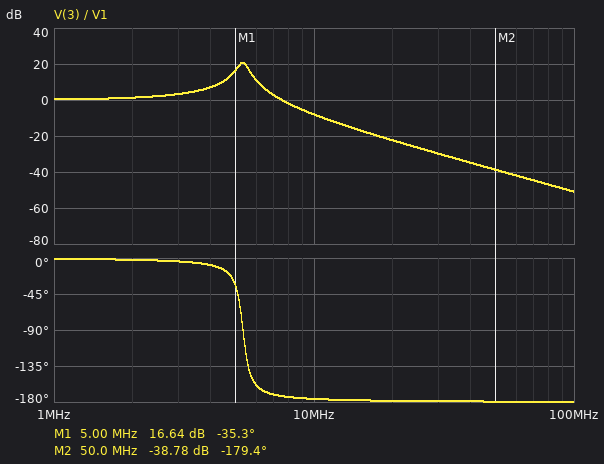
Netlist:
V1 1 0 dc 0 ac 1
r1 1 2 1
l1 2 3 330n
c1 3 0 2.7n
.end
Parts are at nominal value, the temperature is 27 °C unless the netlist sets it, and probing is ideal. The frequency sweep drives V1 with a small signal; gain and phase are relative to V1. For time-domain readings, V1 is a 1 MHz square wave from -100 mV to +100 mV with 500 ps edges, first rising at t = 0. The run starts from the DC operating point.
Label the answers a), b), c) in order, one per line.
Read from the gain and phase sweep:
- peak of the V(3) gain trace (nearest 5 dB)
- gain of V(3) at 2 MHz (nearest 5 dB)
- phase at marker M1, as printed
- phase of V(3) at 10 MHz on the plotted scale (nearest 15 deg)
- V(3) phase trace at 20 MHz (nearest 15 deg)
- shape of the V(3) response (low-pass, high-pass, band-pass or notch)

a) 20 dB
b) 0 dB
c) -35.3 deg
d) -180 deg
e) -180 deg
f) low-pass
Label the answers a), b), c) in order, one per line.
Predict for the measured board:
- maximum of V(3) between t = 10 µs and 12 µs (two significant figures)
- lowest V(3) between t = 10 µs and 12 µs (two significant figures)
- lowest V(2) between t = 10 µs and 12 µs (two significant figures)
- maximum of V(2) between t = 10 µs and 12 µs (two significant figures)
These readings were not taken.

a) 310 mV
b) -310 mV
c) -120 mV
d) 120 mV
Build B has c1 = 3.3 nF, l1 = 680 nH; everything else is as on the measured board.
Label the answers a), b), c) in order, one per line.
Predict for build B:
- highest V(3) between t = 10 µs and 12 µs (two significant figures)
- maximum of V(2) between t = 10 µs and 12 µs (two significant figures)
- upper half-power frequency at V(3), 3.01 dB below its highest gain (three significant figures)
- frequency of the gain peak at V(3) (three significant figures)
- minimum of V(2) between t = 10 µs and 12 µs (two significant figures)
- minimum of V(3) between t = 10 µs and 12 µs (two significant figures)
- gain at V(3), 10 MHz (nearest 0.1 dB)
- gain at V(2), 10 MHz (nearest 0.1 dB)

a) 300 mV
b) 110 mV
c) 3.47 MHz
d) 3.36 MHz
e) -110 mV
f) -300 mV
g) -17.9 dB
h) 0 dB
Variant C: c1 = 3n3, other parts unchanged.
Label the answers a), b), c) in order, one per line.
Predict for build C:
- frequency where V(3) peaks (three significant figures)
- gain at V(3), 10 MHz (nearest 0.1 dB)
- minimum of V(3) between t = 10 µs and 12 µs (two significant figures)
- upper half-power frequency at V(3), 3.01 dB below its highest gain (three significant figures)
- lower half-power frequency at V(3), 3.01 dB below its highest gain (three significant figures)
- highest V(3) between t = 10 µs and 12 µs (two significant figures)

a) 4.81 MHz
b) -10.4 dB
c) -350 mV
d) 5.05 MHz
e) 4.56 MHz
f) 350 mV
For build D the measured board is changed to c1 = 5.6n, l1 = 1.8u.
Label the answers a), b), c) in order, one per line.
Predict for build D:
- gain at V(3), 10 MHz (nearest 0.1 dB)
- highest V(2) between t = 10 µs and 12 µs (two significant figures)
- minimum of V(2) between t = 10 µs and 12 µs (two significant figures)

a) -31.8 dB
b) 110 mV
c) -110 mV
